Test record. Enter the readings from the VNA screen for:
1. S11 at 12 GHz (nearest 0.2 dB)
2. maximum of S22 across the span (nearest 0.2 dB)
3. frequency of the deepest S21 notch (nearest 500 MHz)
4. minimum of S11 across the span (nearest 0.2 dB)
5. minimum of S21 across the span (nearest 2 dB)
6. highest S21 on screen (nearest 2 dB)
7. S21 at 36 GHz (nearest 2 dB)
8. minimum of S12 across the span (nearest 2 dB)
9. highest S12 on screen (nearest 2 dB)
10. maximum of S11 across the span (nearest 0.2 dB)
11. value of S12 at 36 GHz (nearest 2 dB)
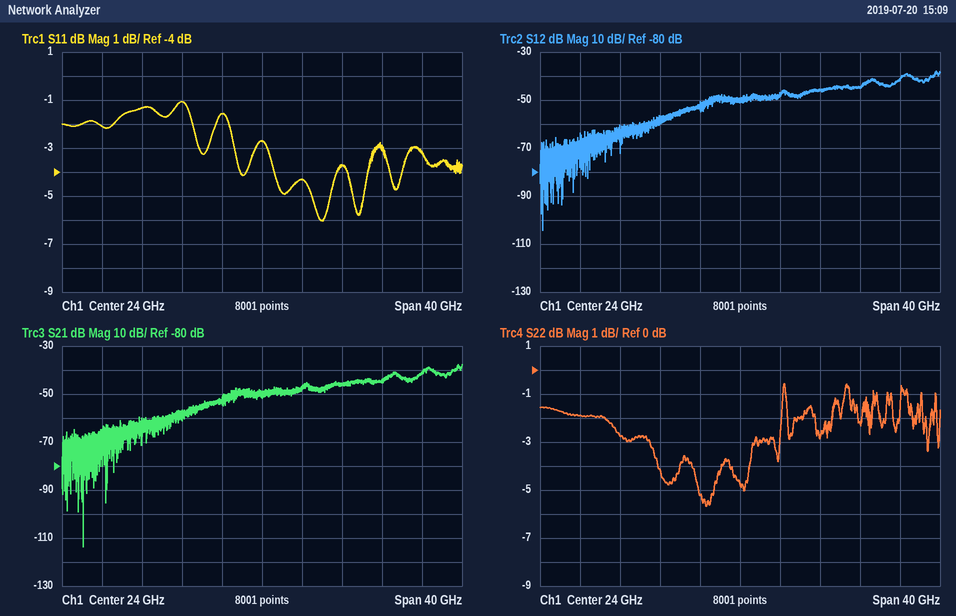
-1.4 dB
-0.6 dB
6.0 GHz
-6.0 dB
-114 dB
-38 dB
-44 dB
-104 dB
-38 dB
-1.0 dB
-44 dB
